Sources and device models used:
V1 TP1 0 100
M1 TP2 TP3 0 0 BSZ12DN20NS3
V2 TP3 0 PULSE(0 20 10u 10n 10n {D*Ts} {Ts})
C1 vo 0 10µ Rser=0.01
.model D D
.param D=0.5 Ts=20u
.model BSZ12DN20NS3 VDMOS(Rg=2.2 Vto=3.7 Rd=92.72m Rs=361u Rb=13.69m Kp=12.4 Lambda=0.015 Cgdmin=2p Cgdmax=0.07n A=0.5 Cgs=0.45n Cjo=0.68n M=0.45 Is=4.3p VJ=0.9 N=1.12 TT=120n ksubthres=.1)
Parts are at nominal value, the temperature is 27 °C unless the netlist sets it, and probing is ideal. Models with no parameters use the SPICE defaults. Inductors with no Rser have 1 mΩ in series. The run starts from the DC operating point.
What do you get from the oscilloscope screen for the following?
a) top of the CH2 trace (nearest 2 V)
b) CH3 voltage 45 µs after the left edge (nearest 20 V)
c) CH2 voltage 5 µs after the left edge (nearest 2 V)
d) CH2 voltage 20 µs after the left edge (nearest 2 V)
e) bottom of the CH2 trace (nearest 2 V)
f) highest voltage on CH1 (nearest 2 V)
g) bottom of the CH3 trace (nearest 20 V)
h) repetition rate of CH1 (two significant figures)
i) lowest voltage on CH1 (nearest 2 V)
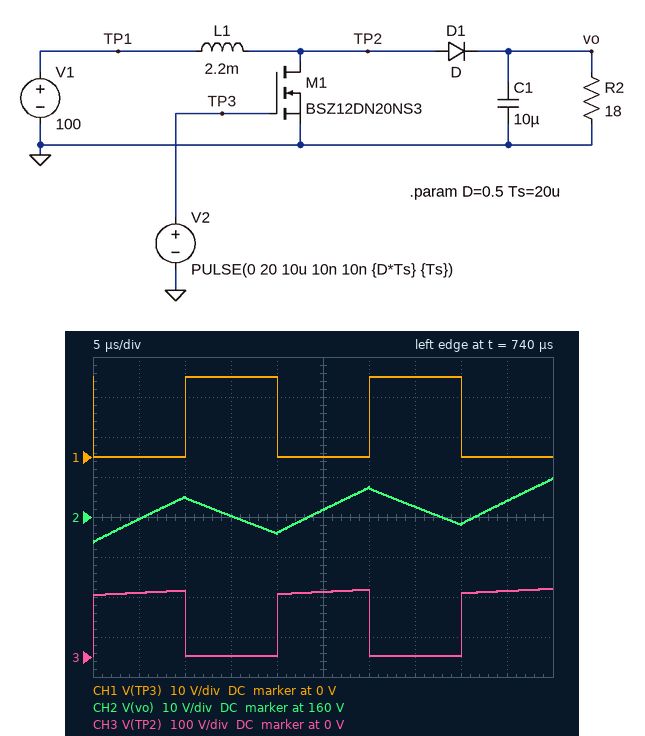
170 V
160 V
160 V
156 V
154 V
20 V
0 V
50 kHz
0 V
